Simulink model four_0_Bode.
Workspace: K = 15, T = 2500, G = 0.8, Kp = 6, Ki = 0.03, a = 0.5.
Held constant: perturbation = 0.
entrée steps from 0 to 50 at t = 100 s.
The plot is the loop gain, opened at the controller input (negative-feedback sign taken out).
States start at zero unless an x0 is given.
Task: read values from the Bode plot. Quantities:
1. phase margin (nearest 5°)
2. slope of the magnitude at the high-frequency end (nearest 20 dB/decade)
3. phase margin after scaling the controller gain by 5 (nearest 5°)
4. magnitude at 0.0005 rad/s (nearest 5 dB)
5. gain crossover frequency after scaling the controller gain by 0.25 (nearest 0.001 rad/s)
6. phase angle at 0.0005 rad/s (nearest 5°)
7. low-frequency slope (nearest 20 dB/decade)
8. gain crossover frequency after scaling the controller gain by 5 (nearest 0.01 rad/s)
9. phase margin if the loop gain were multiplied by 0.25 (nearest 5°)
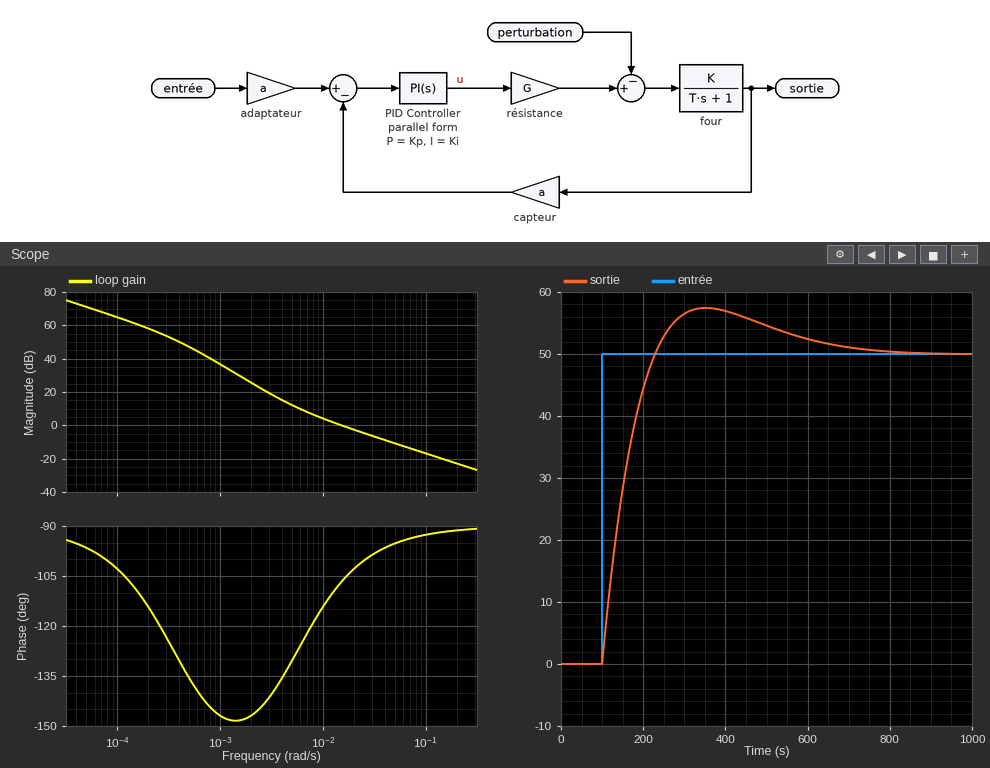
75°
-20 dB/decade
85°
45 dB
0.005 rad/s
-135°
-20 dB/decade
0.07 rad/s
50°
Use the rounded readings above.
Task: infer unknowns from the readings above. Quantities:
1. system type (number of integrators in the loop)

1
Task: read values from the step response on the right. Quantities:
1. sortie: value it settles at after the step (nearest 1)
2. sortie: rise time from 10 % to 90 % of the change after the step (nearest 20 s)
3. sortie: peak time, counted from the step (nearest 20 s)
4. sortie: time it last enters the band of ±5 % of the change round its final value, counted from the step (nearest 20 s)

50
100 s
260 s
500 s
